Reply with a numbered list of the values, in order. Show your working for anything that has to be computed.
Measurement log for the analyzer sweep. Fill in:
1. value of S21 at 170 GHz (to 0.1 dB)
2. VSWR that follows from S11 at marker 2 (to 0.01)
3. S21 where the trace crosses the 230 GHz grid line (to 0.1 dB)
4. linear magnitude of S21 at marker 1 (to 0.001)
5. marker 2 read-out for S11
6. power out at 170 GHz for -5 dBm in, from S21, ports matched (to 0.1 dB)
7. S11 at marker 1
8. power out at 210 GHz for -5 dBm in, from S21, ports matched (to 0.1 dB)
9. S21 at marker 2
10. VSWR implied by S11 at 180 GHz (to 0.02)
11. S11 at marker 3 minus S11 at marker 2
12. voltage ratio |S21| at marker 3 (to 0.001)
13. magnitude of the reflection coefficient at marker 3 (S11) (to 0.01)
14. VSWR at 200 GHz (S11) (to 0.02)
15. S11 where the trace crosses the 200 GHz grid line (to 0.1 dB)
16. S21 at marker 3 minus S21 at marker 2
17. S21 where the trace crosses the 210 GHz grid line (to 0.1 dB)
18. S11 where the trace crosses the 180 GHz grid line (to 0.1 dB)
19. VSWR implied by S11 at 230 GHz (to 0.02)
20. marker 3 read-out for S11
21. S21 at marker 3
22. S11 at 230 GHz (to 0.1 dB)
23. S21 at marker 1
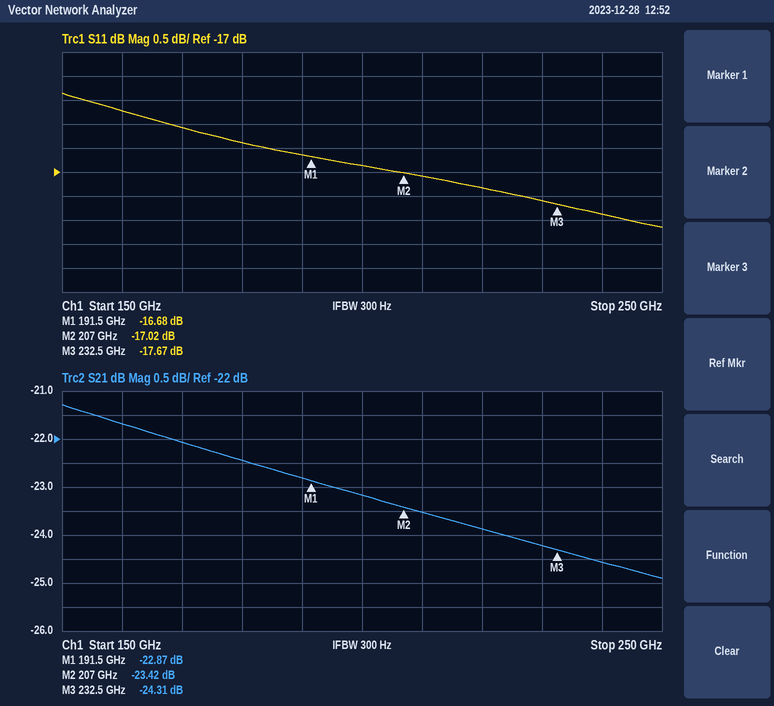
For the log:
1. -22.1 dB
2. (1 + 0.1409)/(1 − 0.1409) ≈ 1.33
3. -24.2 dB
4. 10^(-22.87/20) ≈ 0.072
5. -17.02 dB
6. -5 dBm + (-22.1 dB) = -27.1 dBm
7. -16.68 dB
8. -5 dBm + (-23.5 dB) = -28.5 dBm
9. -23.42 dB
10. |Γ| = 10^(-16.4/20) = 0.1514; VSWR = (1 + 0.1514)/(1 − 0.1514) ≈ 1.36
11. -17.67 − (-17.02) = -0.65 dB
12. 10^(-24.31/20) ≈ 0.061
13. 10^(-17.67/20) ≈ 0.13
14. |Γ| = 10^(-16.9/20) = 0.1429; VSWR = (1 + 0.1429)/(1 − 0.1429) ≈ 1.33, so 1.34 to the nearest 0.02
15. -16.9 dB
16. -24.31 − (-23.42) = -0.89 dB
17. -23.5 dB
18. -16.4 dB
19. |Γ| = 10^(-17.6/20) = 0.1318; VSWR = (1 + 0.1318)/(1 − 0.1318) ≈ 1.30
20. -17.67 dB
21. -24.31 dB
22. -17.6 dB
23. -22.87 dB
